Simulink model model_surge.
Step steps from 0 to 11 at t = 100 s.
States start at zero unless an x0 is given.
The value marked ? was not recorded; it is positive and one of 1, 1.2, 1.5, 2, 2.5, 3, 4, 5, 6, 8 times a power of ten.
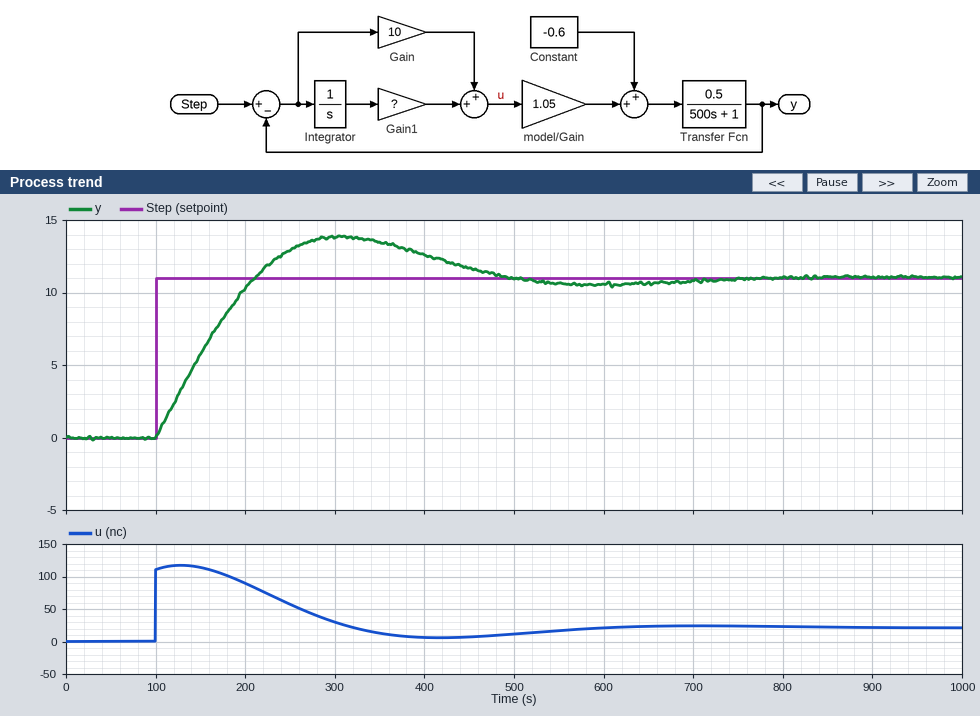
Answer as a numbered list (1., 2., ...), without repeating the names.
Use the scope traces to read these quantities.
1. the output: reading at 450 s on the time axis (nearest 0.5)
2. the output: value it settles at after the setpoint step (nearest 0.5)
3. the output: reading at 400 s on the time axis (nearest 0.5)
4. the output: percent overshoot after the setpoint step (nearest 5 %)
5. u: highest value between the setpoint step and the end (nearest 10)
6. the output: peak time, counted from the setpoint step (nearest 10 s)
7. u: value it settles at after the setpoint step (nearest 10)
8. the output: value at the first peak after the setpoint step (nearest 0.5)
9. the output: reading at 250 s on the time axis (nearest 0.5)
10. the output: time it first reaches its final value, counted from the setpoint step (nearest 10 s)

1. 11.5
2. 11.0
3. 12.5
4. 25 %
5. 120
6. 210 s
7. 20
8. 14.0
9. 13.0
10. 110 s
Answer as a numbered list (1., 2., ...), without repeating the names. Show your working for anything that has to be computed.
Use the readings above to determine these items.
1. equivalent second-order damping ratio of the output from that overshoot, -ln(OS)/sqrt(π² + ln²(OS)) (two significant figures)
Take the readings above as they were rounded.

1. ln(0.25) = -1.386; 1.386 / sqrt(9.870 + 1.922) = 0.40
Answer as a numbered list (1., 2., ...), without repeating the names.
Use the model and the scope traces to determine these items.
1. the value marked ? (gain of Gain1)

1. 0.15
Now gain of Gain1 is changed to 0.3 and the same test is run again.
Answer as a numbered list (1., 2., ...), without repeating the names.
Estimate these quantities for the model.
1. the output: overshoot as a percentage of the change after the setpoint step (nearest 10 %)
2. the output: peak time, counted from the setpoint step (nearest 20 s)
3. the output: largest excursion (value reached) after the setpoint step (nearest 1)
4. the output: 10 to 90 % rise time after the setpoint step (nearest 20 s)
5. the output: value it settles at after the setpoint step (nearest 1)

1. 40 %
2. 160 s
3. 15
4. 60 s
5. 11
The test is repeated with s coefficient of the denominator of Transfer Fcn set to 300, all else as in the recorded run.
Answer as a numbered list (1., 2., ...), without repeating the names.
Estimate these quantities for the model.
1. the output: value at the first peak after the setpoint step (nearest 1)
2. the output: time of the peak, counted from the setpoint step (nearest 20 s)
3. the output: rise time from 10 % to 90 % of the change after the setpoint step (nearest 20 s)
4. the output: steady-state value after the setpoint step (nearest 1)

1. 13
2. 160 s
3. 60 s
4. 11
